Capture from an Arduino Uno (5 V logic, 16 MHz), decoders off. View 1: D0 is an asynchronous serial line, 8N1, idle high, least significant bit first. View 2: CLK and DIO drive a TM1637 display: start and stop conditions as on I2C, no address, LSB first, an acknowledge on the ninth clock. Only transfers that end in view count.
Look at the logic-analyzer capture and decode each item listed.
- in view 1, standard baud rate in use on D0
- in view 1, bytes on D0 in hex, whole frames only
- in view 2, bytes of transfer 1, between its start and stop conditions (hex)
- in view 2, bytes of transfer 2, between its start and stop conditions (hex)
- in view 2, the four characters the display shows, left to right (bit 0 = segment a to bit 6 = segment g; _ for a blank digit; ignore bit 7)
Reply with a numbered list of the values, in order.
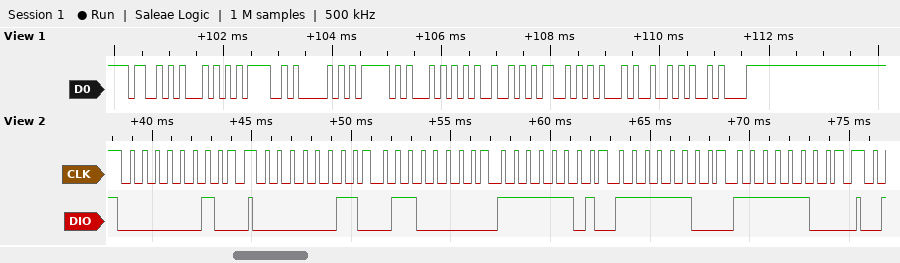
1. 9600 baud
2. 53 54 4F 50 5F 54 49 4D 45 52 0A
3. 40
4. C0 06 BF 3F 3F
5. 1000
